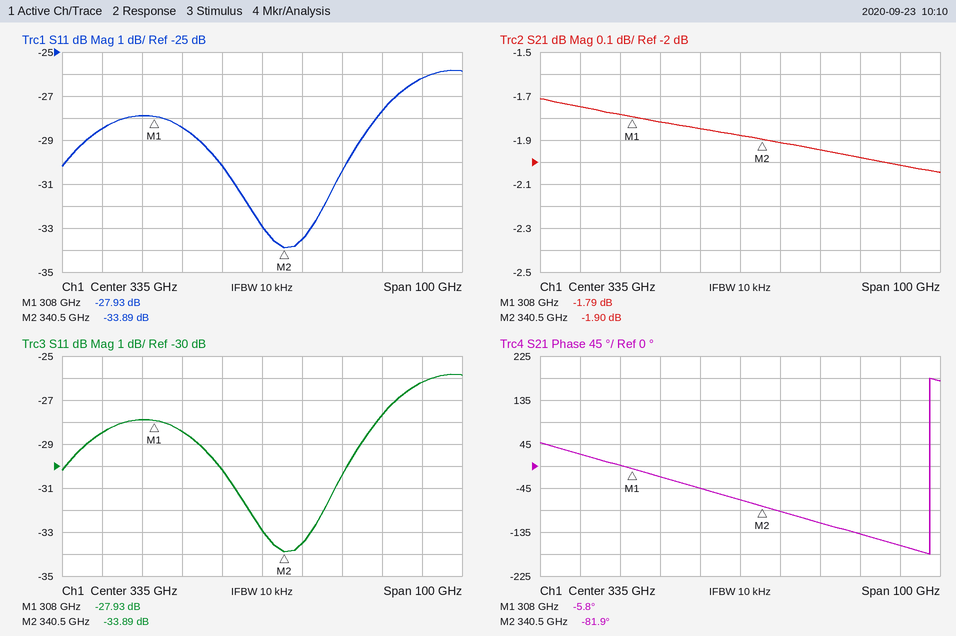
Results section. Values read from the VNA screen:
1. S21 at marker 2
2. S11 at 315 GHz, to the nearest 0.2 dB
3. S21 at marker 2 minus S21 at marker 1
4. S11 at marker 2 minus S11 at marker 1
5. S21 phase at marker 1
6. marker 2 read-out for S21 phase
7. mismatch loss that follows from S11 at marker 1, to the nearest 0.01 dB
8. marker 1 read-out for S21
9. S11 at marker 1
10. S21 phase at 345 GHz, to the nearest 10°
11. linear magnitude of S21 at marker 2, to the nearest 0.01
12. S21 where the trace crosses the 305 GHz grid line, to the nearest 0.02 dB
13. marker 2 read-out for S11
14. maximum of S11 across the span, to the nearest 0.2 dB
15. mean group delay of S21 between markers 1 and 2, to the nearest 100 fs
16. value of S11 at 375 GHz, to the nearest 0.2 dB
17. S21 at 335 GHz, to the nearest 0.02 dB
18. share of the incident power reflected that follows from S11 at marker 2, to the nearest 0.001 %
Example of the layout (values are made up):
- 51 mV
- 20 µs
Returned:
- -1.90 dB
- -28.4 dB
- -0.11 dB
- -5.96 dB
- -5.8°
- -81.9°
- 0.01 dB
- -1.79 dB
- -27.93 dB
- -90°
- 0.80
- -1.78 dB
- -33.89 dB
- -25.8 dB
- 6.5 ps
- -26.2 dB
- -1.88 dB
- 0.041 %
